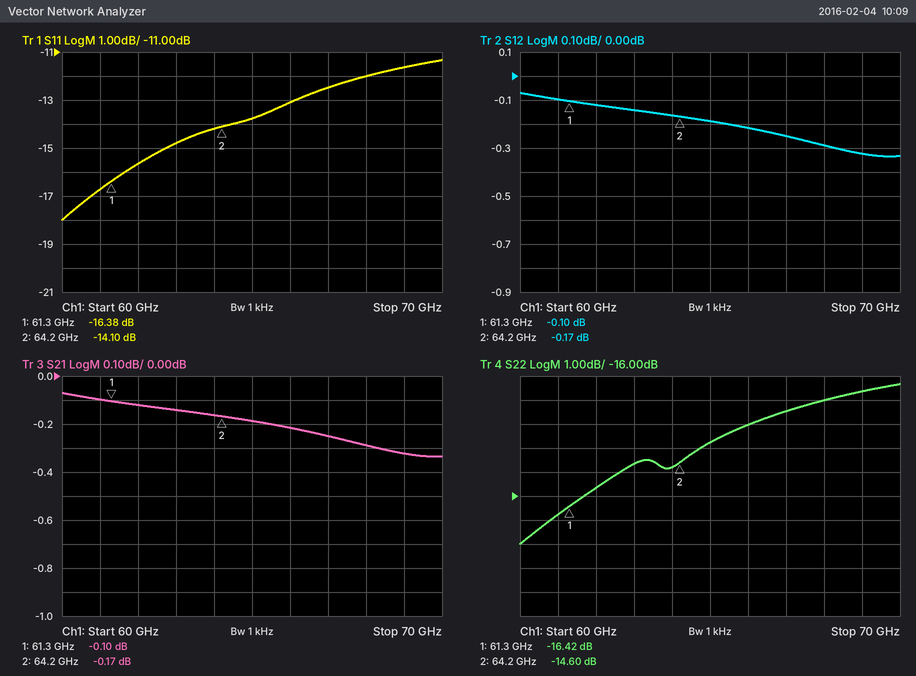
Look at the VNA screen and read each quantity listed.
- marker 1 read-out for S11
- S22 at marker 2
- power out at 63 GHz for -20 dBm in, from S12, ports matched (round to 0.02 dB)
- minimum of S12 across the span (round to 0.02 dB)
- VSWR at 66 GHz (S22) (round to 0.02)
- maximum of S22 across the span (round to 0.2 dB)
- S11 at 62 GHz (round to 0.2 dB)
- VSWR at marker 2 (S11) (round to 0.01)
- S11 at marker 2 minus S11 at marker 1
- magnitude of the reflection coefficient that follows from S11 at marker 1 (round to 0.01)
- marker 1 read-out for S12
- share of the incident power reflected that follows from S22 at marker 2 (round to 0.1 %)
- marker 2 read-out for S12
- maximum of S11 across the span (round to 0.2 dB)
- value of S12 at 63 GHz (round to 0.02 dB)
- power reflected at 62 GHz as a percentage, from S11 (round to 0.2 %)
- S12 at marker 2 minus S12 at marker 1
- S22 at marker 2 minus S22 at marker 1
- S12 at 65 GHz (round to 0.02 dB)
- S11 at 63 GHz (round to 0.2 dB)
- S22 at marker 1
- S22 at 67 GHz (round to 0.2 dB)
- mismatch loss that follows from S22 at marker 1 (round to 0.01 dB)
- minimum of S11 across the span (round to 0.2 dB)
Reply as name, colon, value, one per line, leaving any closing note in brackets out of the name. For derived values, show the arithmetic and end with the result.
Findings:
marker 1 read-out for S11: -16.38 dB
S22 at marker 2: -14.60 dB
power out at 63 GHz for -20 dBm in, from S12, ports matched: -20 dBm + (-0.14 dB) = -20.14 dBm
minimum of S12 across the span: -0.34 dB
VSWR at 66 GHz (S22): |Γ| = 10^(-13/20) = 0.2239; VSWR = (1 + 0.2239)/(1 − 0.2239) ≈ 1.58
maximum of S22 across the span: -11.4 dB
S11 at 62 GHz: -15.6 dB
VSWR at marker 2 (S11): (1 + 0.1972)/(1 − 0.1972) ≈ 1.49
S11 at marker 2 minus S11 at marker 1: -14.1 − (-16.38) = 2.28 dB
magnitude of the reflection coefficient that follows from S11 at marker 1: 10^(-16.38/20) ≈ 0.15
marker 1 read-out for S12: -0.10 dB
share of the incident power reflected that follows from S22 at marker 2: 10^(-14.6/10) ≈ 3.5 %
marker 2 read-out for S12: -0.17 dB
maximum of S11 across the span: -11.4 dB
value of S12 at 63 GHz: -0.14 dB
power reflected at 62 GHz as a percentage, from S11: 10^(-15.6/10) ≈ 2.8 %
S12 at marker 2 minus S12 at marker 1: -0.17 − (-0.1) = -0.07 dB
S22 at marker 2 minus S22 at marker 1: -14.6 − (-16.42) = 1.82 dB
S12 at 65 GHz: -0.18 dB
S11 at 63 GHz: -14.8 dB
S22 at marker 1: -16.42 dB
S22 at 67 GHz: -12.4 dB
mismatch loss that follows from S22 at marker 1: −10 log10(1 − 10^(-16.42/10)) ≈ 0.10 dB
minimum of S11 across the span: -18.0 dB
